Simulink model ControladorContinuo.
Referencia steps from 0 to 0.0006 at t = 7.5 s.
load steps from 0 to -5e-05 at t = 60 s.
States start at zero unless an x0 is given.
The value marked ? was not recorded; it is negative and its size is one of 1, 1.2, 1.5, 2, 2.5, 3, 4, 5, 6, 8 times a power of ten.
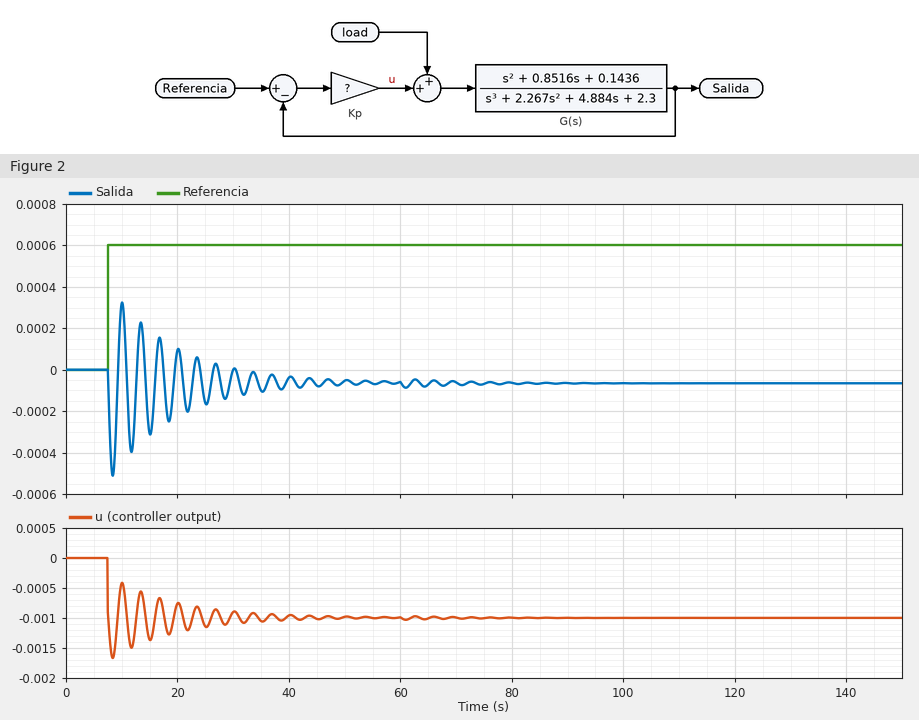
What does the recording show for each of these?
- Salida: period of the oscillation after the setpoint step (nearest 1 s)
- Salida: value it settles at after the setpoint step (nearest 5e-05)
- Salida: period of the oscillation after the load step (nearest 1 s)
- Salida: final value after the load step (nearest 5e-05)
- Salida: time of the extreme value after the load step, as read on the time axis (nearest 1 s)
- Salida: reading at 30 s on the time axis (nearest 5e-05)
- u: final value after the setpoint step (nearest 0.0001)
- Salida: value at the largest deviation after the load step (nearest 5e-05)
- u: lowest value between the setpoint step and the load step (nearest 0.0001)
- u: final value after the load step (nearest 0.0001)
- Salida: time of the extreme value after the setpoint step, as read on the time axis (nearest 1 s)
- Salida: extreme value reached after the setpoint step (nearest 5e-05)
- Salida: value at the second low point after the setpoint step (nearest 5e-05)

3 s
-0.00005
3 s
-0.00005
61 s
0.00000
-0.0010
-0.00010
-0.0017
-0.0010
8 s
-0.00050
-0.00040
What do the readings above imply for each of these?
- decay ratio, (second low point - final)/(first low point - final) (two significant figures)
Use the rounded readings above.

0.78
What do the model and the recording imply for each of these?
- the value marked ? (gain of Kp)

-1.5
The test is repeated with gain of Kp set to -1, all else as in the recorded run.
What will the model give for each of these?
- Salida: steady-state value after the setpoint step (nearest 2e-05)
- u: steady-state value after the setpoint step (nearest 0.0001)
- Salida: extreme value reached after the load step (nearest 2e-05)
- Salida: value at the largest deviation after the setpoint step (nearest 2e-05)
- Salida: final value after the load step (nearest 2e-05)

-0.00004
-0.0006
-0.00006
-0.00028
-0.00004
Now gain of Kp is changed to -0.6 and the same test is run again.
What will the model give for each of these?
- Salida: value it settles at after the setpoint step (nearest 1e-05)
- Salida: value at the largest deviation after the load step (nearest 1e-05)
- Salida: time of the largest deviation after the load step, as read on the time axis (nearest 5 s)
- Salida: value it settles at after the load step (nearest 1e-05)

-0.00002
-0.00004
60 s
-0.00003
